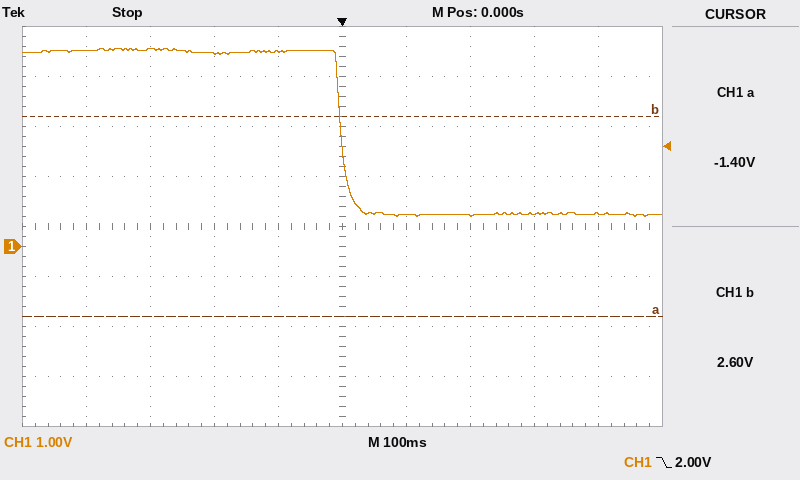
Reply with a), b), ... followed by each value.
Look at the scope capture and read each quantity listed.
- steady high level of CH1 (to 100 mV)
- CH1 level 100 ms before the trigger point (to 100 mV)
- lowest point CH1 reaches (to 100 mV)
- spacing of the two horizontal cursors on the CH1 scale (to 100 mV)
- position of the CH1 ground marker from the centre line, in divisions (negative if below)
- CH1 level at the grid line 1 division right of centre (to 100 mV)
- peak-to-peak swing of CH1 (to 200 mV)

a) 3.9 V
b) 3.9 V
c) 600 mV
d) 4.0 V
e) -0.4 div
f) 600 mV
g) 3.4 V
